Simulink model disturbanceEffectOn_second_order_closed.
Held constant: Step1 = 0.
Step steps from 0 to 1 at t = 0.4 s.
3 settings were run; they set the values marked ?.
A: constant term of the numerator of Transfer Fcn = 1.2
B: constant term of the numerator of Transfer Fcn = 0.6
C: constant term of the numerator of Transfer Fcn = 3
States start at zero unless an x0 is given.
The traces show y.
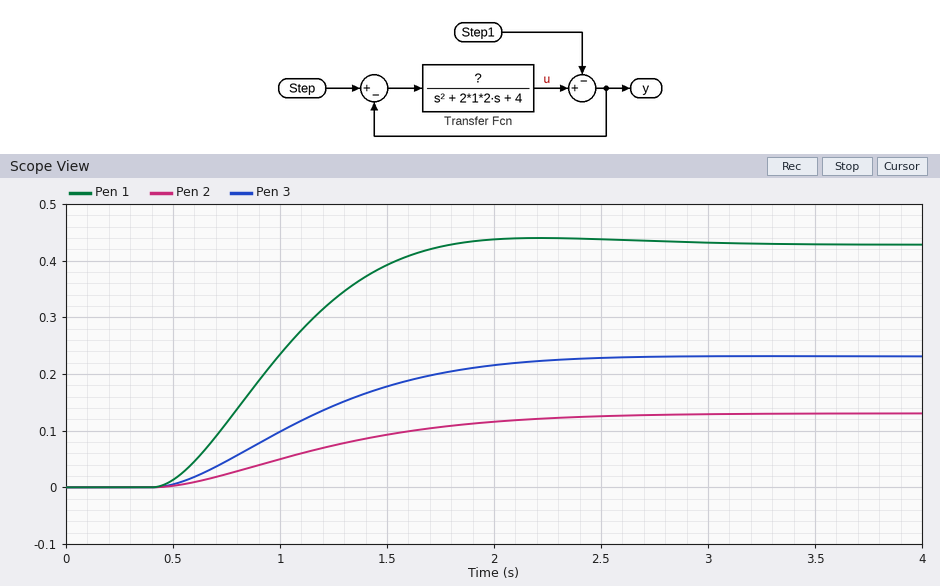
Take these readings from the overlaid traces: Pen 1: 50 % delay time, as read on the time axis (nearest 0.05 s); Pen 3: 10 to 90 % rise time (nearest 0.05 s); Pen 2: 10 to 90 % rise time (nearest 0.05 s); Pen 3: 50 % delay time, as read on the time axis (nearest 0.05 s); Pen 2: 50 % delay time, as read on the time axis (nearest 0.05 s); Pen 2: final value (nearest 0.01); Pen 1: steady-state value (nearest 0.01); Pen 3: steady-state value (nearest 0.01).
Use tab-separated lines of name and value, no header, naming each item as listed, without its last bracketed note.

Pen 1: 50 % delay time, as read on the time axis	0.95 s
Pen 3: 10 to 90 % rise time	1.20 s
Pen 2: 10 to 90 % rise time	1.40 s
Pen 3: 50 % delay time, as read on the time axis	1.10 s
Pen 2: 50 % delay time, as read on the time axis	1.15 s
Pen 2: final value	0.13
Pen 1: steady-state value	0.43
Pen 3: steady-state value	0.23
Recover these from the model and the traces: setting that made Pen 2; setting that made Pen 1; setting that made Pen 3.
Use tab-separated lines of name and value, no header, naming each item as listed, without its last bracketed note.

setting that made Pen 2	B
setting that made Pen 1	C
setting that made Pen 3	A
